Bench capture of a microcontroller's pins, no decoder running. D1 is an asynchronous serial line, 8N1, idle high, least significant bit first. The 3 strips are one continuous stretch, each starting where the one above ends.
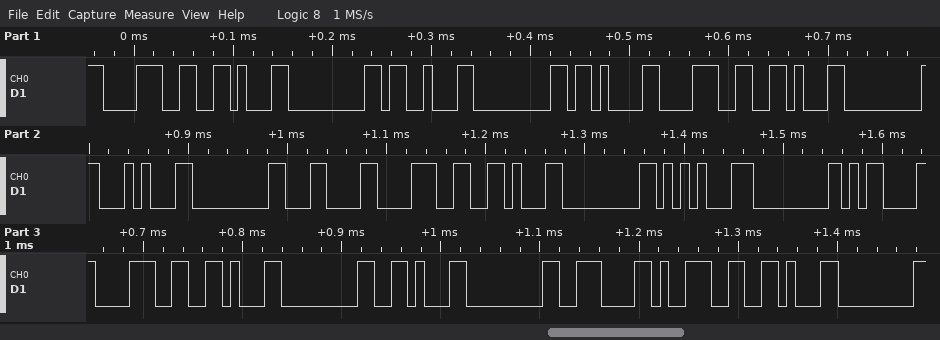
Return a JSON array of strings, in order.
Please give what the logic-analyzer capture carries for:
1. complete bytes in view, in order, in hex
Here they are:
["0x38 0x16 0x00 0x13 0x00 0x0B 0x38 0x16 0x00 0x14 0x00 0x0C 0x38 0x16 0x00 0x15 0x00 0x0D 0x38 0x16 0x00 0x16 0x00 0x0E 0x39 0x16 0x00"]
